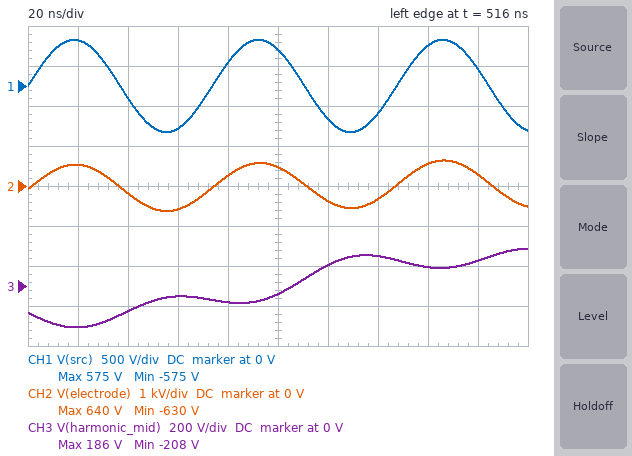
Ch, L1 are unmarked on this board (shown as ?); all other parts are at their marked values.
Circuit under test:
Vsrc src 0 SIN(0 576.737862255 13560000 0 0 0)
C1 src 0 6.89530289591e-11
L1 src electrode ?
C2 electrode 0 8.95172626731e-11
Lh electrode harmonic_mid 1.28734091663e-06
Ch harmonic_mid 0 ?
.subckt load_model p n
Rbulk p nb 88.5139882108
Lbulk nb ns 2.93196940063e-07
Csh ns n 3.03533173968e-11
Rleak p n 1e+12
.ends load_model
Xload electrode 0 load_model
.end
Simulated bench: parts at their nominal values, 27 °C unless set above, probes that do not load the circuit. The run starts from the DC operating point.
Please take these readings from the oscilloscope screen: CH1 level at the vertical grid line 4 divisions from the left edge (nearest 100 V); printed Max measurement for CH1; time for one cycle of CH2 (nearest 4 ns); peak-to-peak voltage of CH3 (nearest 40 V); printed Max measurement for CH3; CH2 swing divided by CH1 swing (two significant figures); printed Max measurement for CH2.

300 V
575 V
72 ns
400 V
186 V
1.1
640 V
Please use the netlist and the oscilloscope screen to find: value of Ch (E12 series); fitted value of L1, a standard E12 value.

1.2 nF
680 nH
